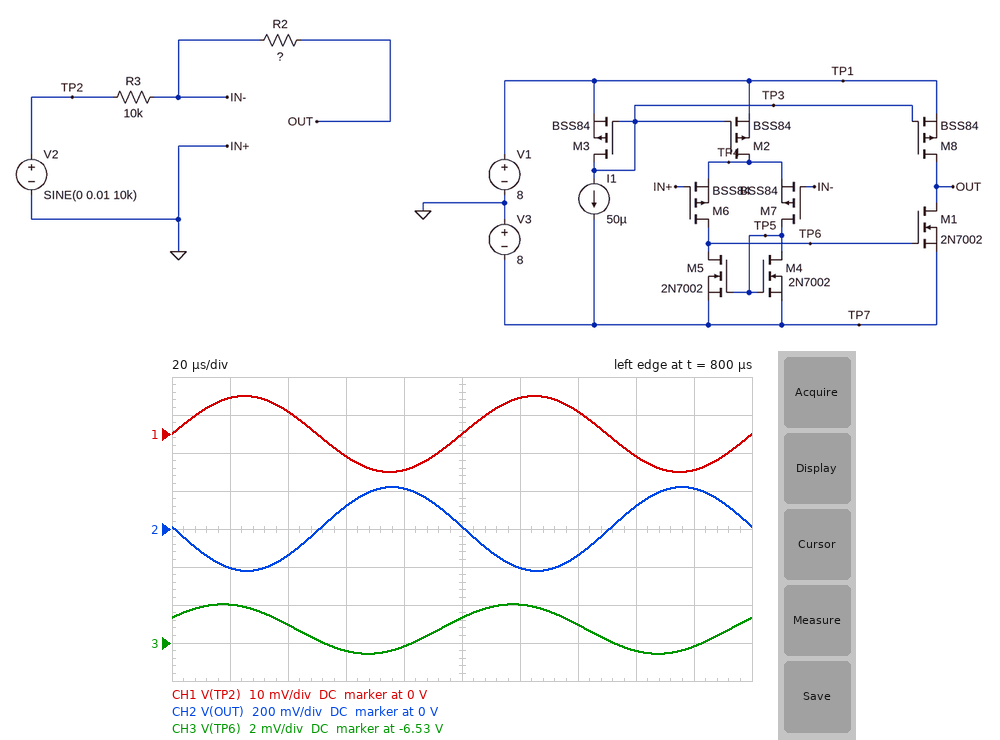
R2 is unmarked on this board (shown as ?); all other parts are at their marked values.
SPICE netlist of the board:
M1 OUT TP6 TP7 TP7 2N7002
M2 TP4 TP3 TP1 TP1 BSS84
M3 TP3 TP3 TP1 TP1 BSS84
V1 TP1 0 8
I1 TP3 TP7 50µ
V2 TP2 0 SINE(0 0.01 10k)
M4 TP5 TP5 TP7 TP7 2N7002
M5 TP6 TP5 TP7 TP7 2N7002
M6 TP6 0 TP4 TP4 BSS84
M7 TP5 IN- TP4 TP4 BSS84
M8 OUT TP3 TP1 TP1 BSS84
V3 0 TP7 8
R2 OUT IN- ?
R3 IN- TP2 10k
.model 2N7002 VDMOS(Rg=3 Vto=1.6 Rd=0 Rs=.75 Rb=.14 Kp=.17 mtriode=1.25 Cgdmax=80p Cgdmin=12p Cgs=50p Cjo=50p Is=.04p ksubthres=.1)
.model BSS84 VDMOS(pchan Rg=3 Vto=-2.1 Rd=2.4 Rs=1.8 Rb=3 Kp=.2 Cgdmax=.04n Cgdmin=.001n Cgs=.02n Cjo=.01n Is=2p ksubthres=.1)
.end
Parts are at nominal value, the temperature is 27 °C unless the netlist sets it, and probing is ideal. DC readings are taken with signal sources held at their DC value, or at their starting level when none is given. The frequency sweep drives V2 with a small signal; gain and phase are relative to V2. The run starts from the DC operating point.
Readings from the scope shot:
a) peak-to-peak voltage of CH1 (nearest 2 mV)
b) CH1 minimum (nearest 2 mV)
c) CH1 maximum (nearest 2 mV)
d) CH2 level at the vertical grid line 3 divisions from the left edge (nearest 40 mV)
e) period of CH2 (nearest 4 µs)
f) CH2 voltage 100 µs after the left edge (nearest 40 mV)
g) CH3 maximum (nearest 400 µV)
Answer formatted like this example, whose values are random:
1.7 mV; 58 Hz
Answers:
20 mV; -10 mV; 10 mV; 120 mV; 100 µs; 0 V; -6.5280 V
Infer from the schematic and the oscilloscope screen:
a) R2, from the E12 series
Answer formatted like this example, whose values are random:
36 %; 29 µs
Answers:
220 kΩ
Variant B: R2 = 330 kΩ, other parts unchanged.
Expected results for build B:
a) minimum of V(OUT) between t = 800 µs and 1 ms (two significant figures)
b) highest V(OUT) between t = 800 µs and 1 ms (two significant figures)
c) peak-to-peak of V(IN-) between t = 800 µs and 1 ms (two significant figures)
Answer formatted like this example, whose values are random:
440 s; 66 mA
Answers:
-330 mV; 330 mV; 1.5 mV
